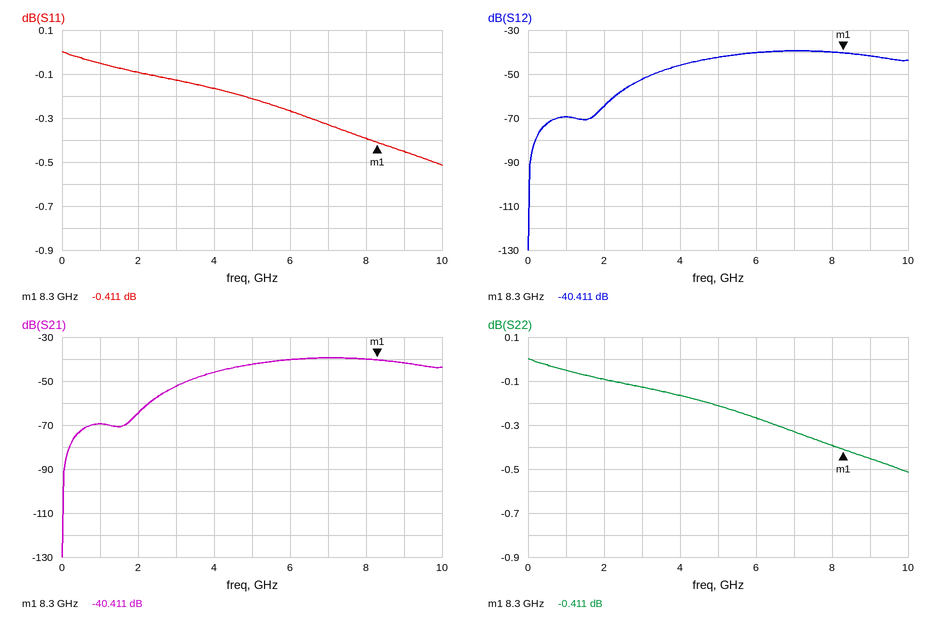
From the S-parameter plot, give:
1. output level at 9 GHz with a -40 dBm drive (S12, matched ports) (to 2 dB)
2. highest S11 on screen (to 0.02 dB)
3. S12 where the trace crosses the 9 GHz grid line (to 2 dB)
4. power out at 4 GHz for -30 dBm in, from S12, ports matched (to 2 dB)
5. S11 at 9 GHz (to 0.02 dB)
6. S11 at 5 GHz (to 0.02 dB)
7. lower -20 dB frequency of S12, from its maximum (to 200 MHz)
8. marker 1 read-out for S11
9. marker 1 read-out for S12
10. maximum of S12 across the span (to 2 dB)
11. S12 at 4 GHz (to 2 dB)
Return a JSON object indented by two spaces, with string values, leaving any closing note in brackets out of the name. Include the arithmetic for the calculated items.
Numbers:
{
  "output level at 9 GHz with a -40 dBm drive (S12, matched ports)": "-40 dBm + (-42 dB) = -82 dBm",
  "highest S11 on screen": "0.00 dB",
  "S12 where the trace crosses the 9 GHz grid line": "-42 dB",
  "power out at 4 GHz for -30 dBm in, from S12, ports matched": "-30 dBm + (-46 dB) = -76 dBm",
  "S11 at 9 GHz": "-0.46 dB",
  "S11 at 5 GHz": "-0.22 dB",
  "lower -20 dB frequency of S12, from its maximum": "2.4 GHz",
  "marker 1 read-out for S11": "-0.411 dB",
  "marker 1 read-out for S12": "-40.411 dB",
  "maximum of S12 across the span": "-40 dB",
  "S12 at 4 GHz": "-46 dB"
}
